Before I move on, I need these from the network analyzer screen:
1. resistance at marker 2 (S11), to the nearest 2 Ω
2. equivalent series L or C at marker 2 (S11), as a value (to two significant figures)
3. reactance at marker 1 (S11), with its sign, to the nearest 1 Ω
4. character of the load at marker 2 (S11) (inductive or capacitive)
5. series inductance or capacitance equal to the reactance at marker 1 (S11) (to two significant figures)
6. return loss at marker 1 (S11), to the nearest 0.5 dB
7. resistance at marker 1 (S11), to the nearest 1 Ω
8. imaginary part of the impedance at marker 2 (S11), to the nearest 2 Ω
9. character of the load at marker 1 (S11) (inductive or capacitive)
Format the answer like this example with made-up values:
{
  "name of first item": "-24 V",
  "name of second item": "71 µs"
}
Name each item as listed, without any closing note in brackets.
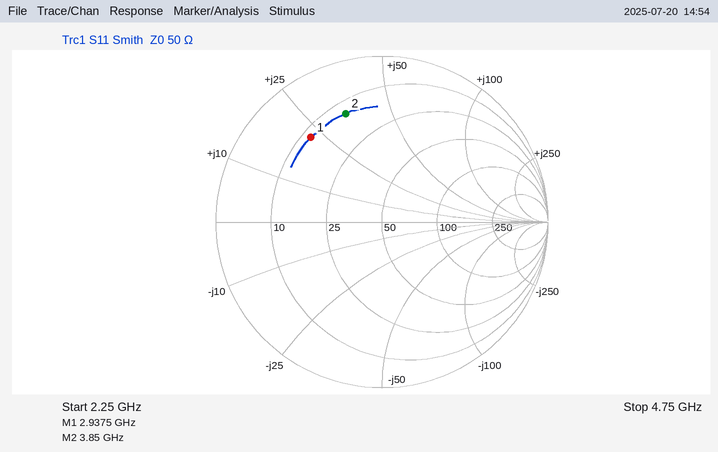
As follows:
{
  "resistance at marker 2 (S11), to the nearest 2 Ω": "14 Ω",
  "equivalent series L or C at marker 2 (S11), as a value": "1.4 nH",
  "reactance at marker 1 (S11), with its sign, to the nearest 1 Ω": "+22 Ω",
  "character of the load at marker 2 (S11)": "inductive",
  "series inductance or capacitance equal to the reactance at marker 1 (S11)": "1.2 nH",
  "return loss at marker 1 (S11), to the nearest 0.5 dB": "3.5 dB",
  "resistance at marker 1 (S11), to the nearest 1 Ω": "12 Ω",
  "imaginary part of the impedance at marker 2 (S11), to the nearest 2 Ω": "+34 Ω",
  "character of the load at marker 1 (S11)": "inductive"
}
